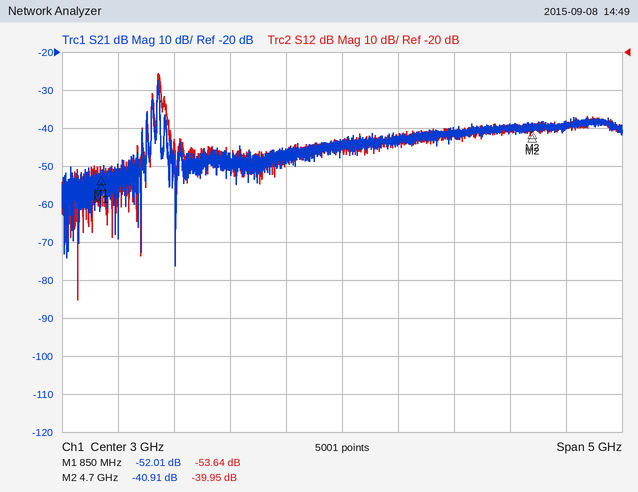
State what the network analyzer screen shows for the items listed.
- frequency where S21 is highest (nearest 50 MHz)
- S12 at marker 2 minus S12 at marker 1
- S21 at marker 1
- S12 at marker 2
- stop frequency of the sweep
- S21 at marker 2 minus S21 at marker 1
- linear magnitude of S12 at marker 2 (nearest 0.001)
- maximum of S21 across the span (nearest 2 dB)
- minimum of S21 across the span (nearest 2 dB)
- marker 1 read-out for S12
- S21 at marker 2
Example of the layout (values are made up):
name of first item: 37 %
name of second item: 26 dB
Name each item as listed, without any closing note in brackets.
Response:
frequency where S21 is highest: 1.35 GHz
S12 at marker 2 minus S12 at marker 1: 13.69 dB
S21 at marker 1: -52.01 dB
S12 at marker 2: -39.95 dB
stop frequency of the sweep: 5.5 GHz
S21 at marker 2 minus S21 at marker 1: 11.10 dB
linear magnitude of S12 at marker 2: 0.010
maximum of S21 across the span: -28 dB
minimum of S21 across the span: -76 dB
marker 1 read-out for S12: -53.64 dB
S21 at marker 2: -40.91 dB
